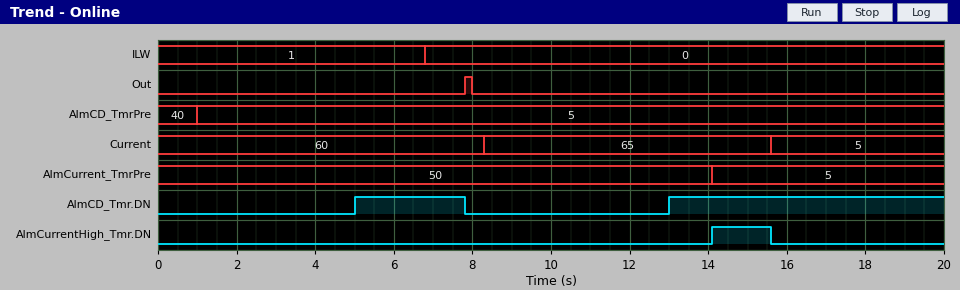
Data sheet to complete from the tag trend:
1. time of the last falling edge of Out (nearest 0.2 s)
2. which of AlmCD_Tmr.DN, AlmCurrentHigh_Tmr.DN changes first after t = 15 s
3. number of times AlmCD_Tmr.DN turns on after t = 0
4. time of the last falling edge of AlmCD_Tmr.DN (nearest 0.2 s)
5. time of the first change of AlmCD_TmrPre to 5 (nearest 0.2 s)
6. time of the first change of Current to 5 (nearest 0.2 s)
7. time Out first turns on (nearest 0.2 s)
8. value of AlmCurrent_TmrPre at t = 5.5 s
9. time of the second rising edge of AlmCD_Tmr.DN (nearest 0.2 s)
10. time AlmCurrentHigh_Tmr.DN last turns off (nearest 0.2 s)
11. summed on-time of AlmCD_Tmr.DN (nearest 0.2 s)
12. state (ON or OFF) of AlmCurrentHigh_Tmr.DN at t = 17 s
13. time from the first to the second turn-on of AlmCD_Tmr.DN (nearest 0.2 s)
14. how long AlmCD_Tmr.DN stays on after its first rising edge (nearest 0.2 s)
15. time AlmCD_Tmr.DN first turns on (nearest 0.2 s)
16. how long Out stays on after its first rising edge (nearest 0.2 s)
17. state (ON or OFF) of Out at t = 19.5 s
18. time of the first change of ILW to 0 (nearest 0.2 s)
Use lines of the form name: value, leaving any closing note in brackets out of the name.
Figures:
time of the last falling edge of Out: 8.0 s
which of AlmCD_Tmr.DN, AlmCurrentHigh_Tmr.DN changes first after t = 15 s: AlmCurrentHigh_Tmr.DN
number of times AlmCD_Tmr.DN turns on after t = 0: 2
time of the last falling edge of AlmCD_Tmr.DN: 7.8 s
time of the first change of AlmCD_TmrPre to 5: 1.0 s
time of the first change of Current to 5: 15.6 s
time Out first turns on: 7.8 s
value of AlmCurrent_TmrPre at t = 5.5 s: 50
time of the second rising edge of AlmCD_Tmr.DN: 13.0 s
time AlmCurrentHigh_Tmr.DN last turns off: 15.6 s
summed on-time of AlmCD_Tmr.DN: 9.8 s
state (ON or OFF) of AlmCurrentHigh_Tmr.DN at t = 17 s: OFF
time from the first to the second turn-on of AlmCD_Tmr.DN: 8.0 s
how long AlmCD_Tmr.DN stays on after its first rising edge: 2.8 s
time AlmCD_Tmr.DN first turns on: 5.0 s
how long Out stays on after its first rising edge: 0.2 s
state (ON or OFF) of Out at t = 19.5 s: OFF
time of the first change of ILW to 0: 6.8 s
